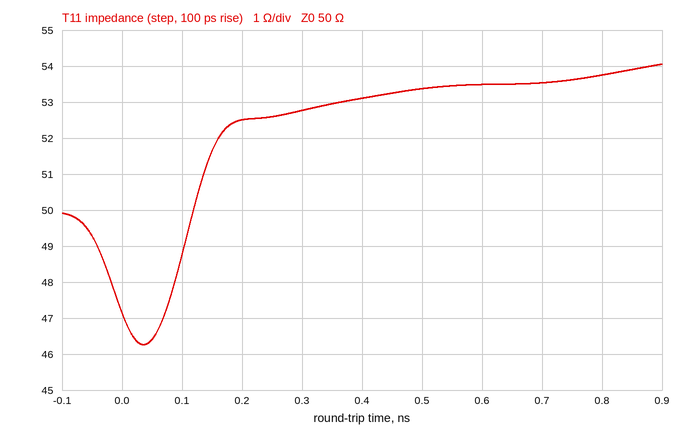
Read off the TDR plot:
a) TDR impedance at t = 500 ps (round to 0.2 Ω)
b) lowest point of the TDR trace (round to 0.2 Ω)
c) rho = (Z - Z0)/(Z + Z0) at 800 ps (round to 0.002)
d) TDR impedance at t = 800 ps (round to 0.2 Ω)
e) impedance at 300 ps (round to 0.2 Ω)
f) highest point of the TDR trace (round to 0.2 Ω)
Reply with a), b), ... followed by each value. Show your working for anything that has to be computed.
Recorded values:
a) 53.4 Ω
b) 46.2 Ω
c) (53.8 − 50)/(53.8 + 50) ≈ +0.0366, so +0.036 to the nearest 0.002
d) 53.8 Ω
e) 52.8 Ω
f) 54.0 Ω
